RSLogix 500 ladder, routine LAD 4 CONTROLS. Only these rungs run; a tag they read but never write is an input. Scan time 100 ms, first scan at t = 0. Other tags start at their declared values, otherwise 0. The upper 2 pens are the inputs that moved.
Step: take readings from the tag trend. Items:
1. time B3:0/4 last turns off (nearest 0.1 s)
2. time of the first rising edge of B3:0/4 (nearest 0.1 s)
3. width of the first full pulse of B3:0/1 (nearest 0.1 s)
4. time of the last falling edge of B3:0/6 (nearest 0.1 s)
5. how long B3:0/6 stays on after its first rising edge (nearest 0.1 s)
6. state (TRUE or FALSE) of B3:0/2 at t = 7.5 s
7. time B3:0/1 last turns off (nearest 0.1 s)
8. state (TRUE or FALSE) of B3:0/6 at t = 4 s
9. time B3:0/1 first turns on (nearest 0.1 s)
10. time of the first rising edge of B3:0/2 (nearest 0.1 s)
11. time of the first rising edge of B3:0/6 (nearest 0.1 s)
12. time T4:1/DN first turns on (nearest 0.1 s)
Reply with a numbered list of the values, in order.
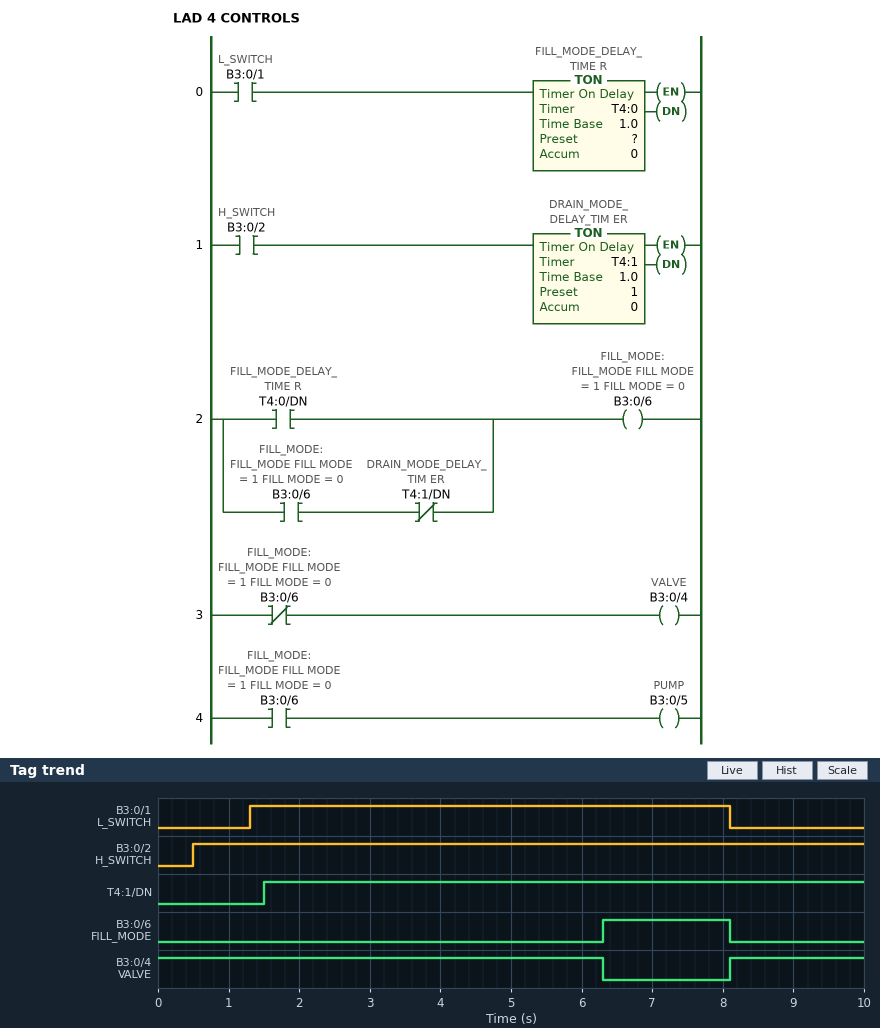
1. 6.3 s
2. 8.1 s
3. 6.8 s
4. 8.1 s
5. 1.8 s
6. TRUE
7. 8.1 s
8. FALSE
9. 1.3 s
10. 0.5 s
11. 6.3 s
12. 1.5 s
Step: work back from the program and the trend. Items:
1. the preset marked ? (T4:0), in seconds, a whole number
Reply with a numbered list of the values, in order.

1. 5 s
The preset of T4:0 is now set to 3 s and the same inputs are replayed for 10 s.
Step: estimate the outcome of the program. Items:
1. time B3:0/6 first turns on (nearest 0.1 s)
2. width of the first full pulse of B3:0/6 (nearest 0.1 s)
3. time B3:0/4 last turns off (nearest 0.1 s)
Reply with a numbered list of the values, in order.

1. 4.3 s
2. 3.8 s
3. 4.3 s
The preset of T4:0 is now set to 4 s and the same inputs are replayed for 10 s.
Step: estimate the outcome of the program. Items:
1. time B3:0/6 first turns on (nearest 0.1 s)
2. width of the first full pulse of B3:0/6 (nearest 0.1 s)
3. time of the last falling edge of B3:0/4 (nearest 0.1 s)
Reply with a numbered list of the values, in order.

1. 5.3 s
2. 2.8 s
3. 5.3 s
